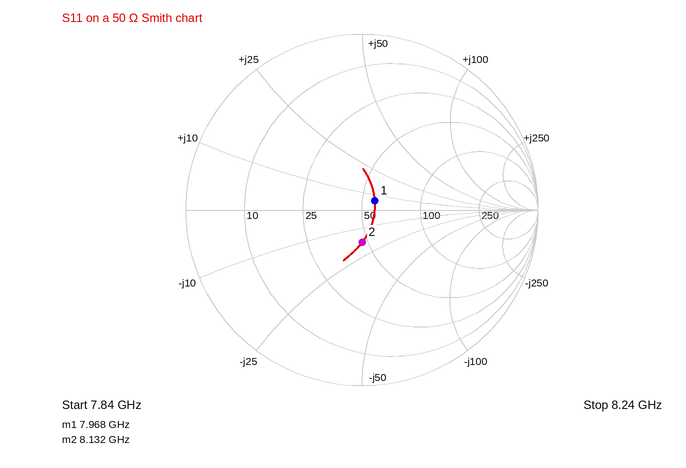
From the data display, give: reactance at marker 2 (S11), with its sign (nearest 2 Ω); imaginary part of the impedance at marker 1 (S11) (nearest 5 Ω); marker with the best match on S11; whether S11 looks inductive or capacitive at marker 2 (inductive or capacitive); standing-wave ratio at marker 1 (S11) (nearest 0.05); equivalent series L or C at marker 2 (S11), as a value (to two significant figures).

-18 Ω
+5 Ω
marker 1
capacitive
1.20
1.1 pF
